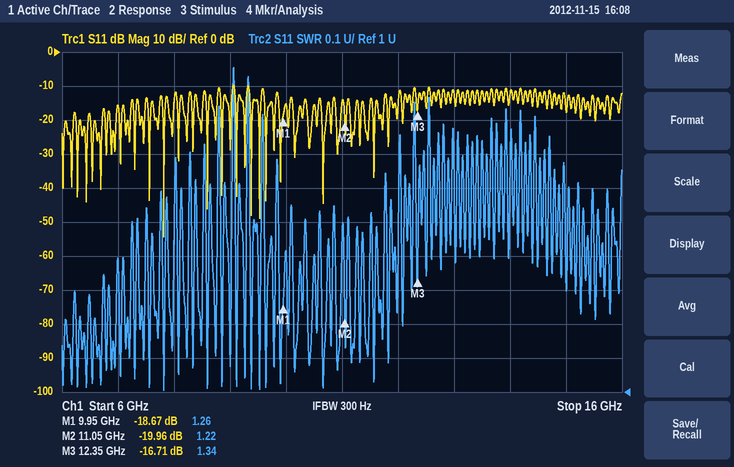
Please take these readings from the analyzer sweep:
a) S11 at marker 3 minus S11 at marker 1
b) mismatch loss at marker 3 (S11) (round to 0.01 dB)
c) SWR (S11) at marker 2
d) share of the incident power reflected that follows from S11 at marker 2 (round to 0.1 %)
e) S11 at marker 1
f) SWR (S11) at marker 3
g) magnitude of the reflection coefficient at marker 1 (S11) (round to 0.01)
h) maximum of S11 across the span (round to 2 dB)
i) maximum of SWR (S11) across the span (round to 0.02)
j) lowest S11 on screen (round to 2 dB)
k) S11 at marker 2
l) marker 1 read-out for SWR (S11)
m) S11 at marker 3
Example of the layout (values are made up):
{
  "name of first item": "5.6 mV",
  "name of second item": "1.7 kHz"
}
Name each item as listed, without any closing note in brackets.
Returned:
{
  "S11 at marker 3 minus S11 at marker 1": "1.96 dB",
  "mismatch loss at marker 3 (S11)": "0.09 dB",
  "SWR (S11) at marker 2": "1.22",
  "share of the incident power reflected that follows from S11 at marker 2": "1.0 %",
  "S11 at marker 1": "-18.67 dB",
  "SWR (S11) at marker 3": "1.34",
  "magnitude of the reflection coefficient at marker 1 (S11)": "0.12",
  "maximum of S11 across the span": "-10 dB",
  "maximum of SWR (S11) across the span": "1.96",
  "lowest S11 on screen": "-54 dB",
  "S11 at marker 2": "-19.96 dB",
  "marker 1 read-out for SWR": "1.26",
  "S11 at marker 3": "-16.71 dB"
}
